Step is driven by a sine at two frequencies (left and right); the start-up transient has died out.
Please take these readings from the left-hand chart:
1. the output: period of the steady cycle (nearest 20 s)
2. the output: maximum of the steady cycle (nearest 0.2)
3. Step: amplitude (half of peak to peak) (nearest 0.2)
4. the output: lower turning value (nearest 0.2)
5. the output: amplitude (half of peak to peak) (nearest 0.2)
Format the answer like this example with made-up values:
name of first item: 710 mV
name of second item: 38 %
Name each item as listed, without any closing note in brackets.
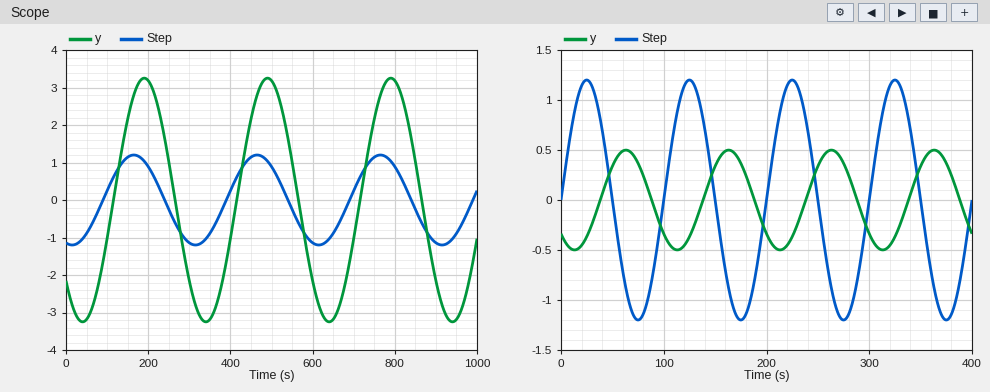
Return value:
the output: period of the steady cycle: 300 s
the output: maximum of the steady cycle: 3.2
Step: amplitude (half of peak to peak): 1.2
the output: lower turning value: -3.2
the output: amplitude (half of peak to peak): 3.2
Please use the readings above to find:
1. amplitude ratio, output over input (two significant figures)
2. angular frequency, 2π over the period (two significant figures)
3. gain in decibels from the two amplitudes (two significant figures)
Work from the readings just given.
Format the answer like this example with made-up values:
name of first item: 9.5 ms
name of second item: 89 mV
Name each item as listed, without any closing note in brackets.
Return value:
amplitude ratio, output over input: 2.7
angular frequency, 2π over the period: 0.021 rad/s
gain in decibels from the two amplitudes: 8.5 dB
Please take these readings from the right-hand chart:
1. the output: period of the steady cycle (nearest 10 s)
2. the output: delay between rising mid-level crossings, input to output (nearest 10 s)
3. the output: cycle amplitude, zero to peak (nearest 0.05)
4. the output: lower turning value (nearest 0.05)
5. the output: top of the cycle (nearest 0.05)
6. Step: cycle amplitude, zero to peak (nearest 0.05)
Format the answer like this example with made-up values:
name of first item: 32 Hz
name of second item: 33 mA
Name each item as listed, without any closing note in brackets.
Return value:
the output: period of the steady cycle: 100 s
the output: delay between rising mid-level crossings, input to output: 40 s
the output: cycle amplitude, zero to peak: 0.50
the output: lower turning value: -0.50
the output: top of the cycle: 0.50
Step: cycle amplitude, zero to peak: 1.20
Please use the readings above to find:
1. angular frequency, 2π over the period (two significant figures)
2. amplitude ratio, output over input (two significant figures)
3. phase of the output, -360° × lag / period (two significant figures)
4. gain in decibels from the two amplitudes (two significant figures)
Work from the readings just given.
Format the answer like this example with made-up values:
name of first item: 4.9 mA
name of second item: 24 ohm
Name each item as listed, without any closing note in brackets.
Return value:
angular frequency, 2π over the period: 0.063 rad/s
amplitude ratio, output over input: 0.42
phase of the output, -360° × lag / period: -140°
gain in decibels from the two amplitudes: -7.6 dB
